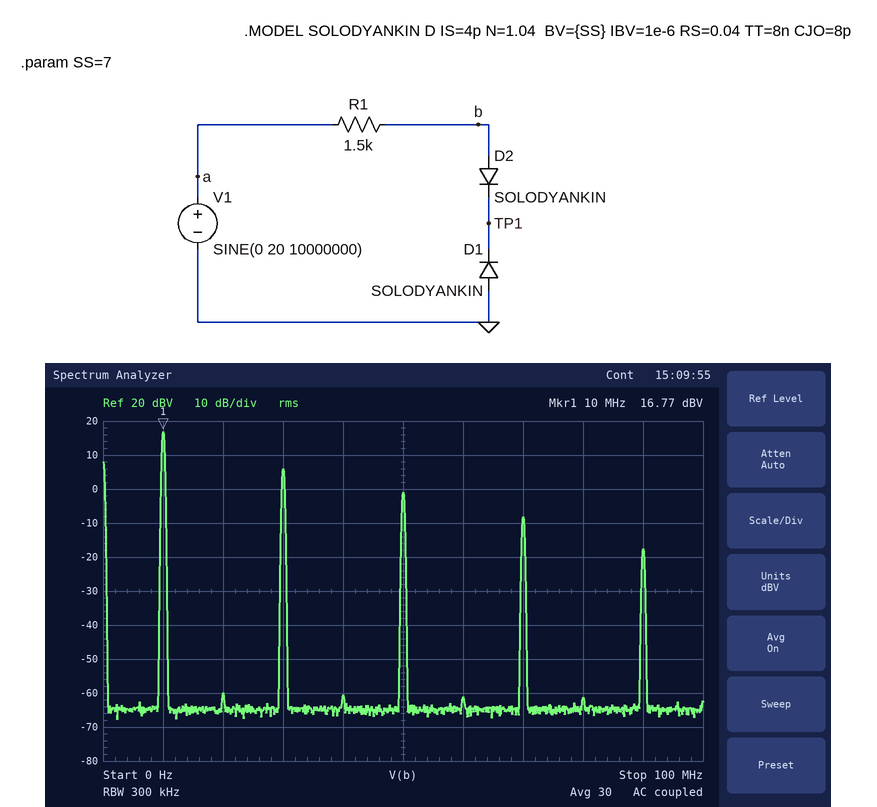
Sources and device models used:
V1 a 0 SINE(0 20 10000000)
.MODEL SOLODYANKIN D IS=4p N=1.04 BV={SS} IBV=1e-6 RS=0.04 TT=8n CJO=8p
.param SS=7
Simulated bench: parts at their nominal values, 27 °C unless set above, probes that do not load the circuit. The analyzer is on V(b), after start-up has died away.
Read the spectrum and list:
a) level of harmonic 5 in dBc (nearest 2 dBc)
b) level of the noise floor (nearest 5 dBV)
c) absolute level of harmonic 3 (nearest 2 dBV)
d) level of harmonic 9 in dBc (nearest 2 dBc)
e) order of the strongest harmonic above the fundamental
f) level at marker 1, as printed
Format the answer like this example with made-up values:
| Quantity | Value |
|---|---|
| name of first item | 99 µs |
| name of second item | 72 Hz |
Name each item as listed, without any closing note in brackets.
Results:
| Quantity | Value |
|---|---|
| level of harmonic 5 in dBc | -18 dBc |
| level of the noise floor | -65 dBV |
| absolute level of harmonic 3 | 6 dBV |
| level of harmonic 9 in dBc | -34 dBc |
| order of the strongest harmonic above the fundamental | 3 |
| level at marker 1, as printed | 16.77 dBV |
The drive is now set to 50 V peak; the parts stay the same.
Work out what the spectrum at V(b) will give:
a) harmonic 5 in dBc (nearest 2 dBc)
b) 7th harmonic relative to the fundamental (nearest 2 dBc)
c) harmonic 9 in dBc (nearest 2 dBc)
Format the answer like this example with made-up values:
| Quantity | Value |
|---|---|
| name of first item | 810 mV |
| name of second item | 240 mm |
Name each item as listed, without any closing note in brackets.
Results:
| Quantity | Value |
|---|---|
| harmonic 5 in dBc | -14 dBc |
| 7th harmonic relative to the fundamental | -18 dBc |
| harmonic 9 in dBc | -20 dBc |
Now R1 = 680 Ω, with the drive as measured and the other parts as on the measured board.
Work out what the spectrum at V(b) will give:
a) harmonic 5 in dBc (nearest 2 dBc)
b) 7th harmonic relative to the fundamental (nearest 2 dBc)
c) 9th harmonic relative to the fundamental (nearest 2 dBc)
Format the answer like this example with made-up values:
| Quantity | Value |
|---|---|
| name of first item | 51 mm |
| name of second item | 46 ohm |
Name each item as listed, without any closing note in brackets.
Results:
| Quantity | Value |
|---|---|
| harmonic 5 in dBc | -16 dBc |
| 7th harmonic relative to the fundamental | -22 dBc |
| 9th harmonic relative to the fundamental | -26 dBc |
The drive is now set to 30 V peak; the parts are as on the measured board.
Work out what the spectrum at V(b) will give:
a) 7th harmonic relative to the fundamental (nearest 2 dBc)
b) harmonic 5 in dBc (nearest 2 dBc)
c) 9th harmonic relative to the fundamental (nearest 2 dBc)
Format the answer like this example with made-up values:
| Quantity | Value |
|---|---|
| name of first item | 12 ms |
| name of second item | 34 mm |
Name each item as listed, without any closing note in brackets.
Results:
| Quantity | Value |
|---|---|
| 7th harmonic relative to the fundamental | -20 dBc |
| harmonic 5 in dBc | -16 dBc |
| 9th harmonic relative to the fundamental | -24 dBc |
